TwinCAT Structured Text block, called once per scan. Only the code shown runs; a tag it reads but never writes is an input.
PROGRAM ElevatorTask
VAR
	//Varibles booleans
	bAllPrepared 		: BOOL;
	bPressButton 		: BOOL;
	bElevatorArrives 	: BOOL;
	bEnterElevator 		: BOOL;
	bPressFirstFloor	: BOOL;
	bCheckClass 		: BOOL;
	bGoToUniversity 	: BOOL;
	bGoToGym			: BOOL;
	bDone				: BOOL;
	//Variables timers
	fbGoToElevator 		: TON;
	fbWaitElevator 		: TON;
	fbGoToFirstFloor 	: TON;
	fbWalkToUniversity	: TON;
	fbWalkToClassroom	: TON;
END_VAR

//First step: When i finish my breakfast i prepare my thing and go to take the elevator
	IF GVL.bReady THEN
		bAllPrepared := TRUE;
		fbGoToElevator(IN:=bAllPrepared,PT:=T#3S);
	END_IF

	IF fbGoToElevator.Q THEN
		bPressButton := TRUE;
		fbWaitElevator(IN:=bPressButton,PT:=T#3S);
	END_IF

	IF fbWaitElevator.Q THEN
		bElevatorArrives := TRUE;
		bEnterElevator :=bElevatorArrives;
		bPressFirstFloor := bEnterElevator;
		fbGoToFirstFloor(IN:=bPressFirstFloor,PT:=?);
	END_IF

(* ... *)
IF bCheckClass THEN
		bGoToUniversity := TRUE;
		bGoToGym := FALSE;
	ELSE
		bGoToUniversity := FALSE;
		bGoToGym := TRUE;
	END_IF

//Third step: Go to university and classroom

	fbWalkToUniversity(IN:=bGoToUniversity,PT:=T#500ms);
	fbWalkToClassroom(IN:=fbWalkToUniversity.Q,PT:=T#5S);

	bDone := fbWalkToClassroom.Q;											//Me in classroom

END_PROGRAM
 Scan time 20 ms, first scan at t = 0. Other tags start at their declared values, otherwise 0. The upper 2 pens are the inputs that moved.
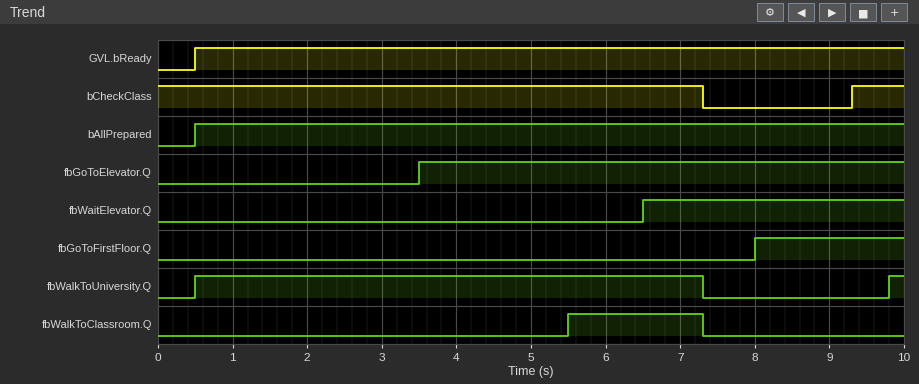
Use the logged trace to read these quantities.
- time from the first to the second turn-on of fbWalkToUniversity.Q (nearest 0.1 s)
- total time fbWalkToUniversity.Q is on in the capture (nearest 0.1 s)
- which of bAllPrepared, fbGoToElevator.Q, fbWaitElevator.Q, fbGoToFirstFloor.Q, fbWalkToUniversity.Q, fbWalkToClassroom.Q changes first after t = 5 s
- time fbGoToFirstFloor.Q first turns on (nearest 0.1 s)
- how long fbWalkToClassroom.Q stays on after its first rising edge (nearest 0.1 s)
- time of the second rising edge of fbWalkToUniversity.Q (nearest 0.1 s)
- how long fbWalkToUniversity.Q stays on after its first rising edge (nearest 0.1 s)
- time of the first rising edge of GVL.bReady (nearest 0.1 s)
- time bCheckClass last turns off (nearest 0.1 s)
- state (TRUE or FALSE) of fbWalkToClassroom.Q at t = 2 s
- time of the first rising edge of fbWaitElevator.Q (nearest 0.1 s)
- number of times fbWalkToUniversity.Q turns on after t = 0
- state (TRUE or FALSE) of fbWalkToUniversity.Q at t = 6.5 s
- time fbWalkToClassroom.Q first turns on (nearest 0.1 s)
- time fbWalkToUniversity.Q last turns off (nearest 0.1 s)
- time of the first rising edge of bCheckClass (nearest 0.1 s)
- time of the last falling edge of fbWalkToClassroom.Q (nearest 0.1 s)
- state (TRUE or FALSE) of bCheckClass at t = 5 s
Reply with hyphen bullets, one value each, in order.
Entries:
- 9.3 s
- 7.0 s
- fbWalkToClassroom.Q
- 8.0 s
- 1.8 s
- 9.8 s
- 6.8 s
- 0.5 s
- 7.3 s
- FALSE
- 6.5 s
- 2
- TRUE
- 5.5 s
- 7.3 s
- 9.3 s
- 7.3 s
- TRUE
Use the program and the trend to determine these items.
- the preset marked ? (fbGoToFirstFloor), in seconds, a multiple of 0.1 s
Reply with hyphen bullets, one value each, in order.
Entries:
- 1.5 s
